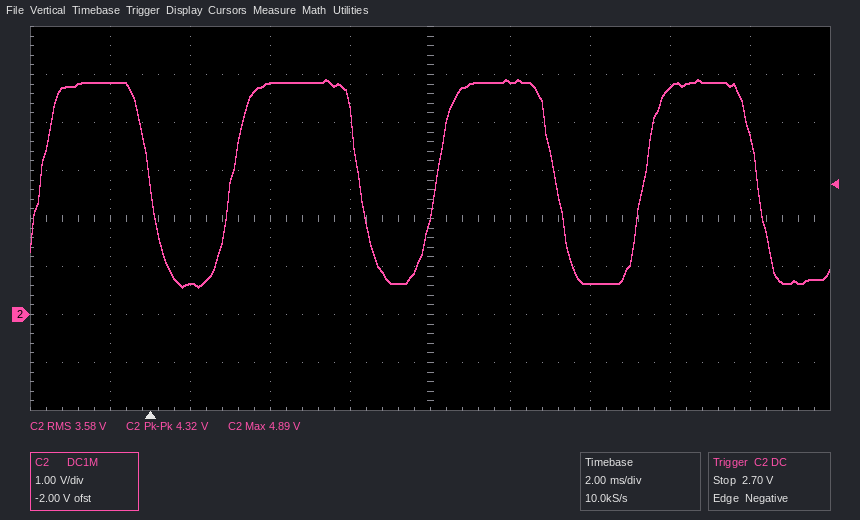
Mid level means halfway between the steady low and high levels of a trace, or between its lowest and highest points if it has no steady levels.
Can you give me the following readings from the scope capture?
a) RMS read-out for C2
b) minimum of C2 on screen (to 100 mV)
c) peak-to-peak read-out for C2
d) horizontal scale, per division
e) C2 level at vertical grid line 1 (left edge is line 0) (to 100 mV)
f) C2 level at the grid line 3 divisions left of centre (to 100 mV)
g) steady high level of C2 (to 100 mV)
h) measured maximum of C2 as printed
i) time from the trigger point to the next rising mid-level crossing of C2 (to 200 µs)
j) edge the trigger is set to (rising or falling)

3.58 V
600 mV
4.32 V
2 ms
4.8 V
600 mV
4.8 V
4.89 V
2.0 ms
falling
